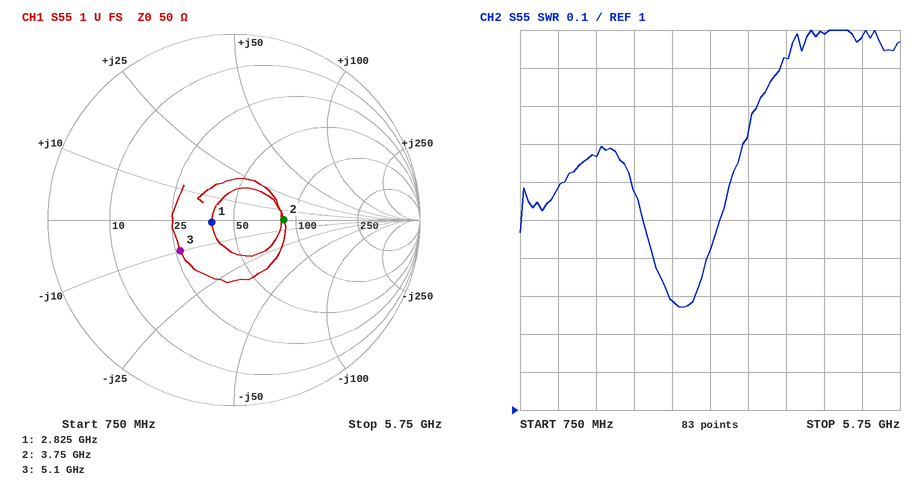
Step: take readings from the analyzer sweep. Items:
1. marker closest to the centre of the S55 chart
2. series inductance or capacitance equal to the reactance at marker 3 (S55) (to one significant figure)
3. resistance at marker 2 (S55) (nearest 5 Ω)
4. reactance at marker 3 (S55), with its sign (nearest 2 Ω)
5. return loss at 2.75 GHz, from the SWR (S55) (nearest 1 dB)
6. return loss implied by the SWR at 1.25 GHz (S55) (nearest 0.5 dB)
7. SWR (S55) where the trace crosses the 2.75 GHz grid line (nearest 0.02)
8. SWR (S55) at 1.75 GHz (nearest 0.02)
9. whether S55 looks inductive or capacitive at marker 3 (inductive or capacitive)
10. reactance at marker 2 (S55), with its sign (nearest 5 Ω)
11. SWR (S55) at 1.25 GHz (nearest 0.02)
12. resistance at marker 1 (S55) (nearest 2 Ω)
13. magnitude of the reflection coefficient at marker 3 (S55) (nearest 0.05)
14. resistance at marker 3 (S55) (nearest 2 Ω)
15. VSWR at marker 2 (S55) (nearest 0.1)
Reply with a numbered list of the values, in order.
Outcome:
1. marker 1
2. 3 pF
3. 85 Ω
4. -10 Ω
5. 18 dB
6. 13.0 dB
7. 1.28
8. 1.66
9. capacitive
10. 0 Ω
11. 1.58
12. 40 Ω
13. 0.35
14. 26 Ω
15. 1.7
